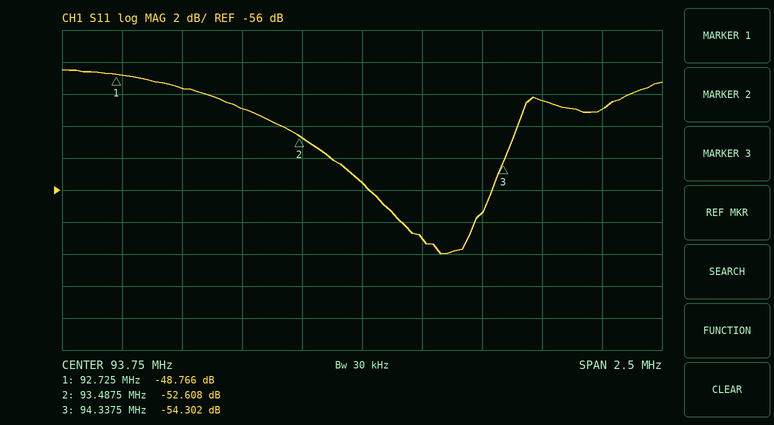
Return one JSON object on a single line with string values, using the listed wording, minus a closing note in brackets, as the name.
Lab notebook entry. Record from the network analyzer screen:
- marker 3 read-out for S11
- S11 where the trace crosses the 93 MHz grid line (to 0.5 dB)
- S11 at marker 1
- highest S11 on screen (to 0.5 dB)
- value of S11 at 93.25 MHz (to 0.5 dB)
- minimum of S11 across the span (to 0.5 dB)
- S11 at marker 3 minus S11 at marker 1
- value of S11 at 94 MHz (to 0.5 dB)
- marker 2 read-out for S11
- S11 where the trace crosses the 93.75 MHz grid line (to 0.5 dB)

{"marker 3 read-out for S11": "-54.302 dB", "S11 where the trace crosses the 93 MHz grid line": "-49.5 dB", "S11 at marker 1": "-48.766 dB", "highest S11 on screen": "-48.5 dB", "value of S11 at 93.25 MHz": "-51.0 dB", "minimum of S11 across the span": "-60.0 dB", "S11 at marker 3 minus S11 at marker 1": "-5.536 dB", "value of S11 at 94 MHz": "-59.0 dB", "marker 2 read-out for S11": "-52.608 dB", "S11 where the trace crosses the 93.75 MHz grid line": "-55.5 dB"}
